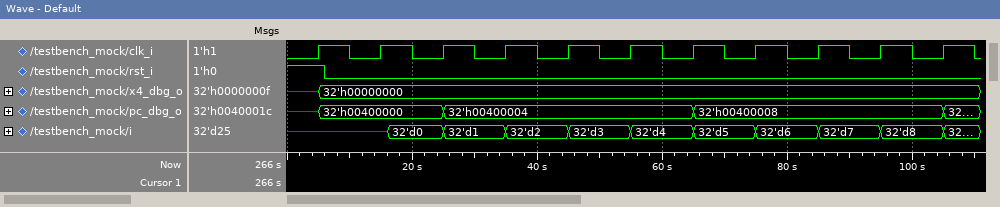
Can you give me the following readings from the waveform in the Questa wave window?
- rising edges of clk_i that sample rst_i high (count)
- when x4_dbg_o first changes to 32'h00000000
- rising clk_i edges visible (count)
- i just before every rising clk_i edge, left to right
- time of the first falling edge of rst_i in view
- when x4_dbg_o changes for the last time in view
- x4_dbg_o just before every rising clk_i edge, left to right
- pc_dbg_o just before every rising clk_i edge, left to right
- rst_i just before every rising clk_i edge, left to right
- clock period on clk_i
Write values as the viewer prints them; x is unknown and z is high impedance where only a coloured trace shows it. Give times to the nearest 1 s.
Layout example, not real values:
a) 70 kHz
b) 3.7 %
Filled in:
a) 1
b) 5 s
c) 11
d) x, x, 32'd0, 32'd1, 32'd2, 32'd3, 32'd4, 32'd5, 32'd6, 32'd7, 32'd8
e) 6 s
f) 5 s
g) x, 32'h00000000, 32'h00000000, 32'h00000000, 32'h00000000, 32'h00000000, 32'h00000000, 32'h00000000, 32'h00000000, 32'h00000000, 32'h00000000
h) x, 32'h00400000, 32'h00400000, 32'h00400004, 32'h00400004, 32'h00400004, 32'h00400004, 32'h00400008, 32'h00400008, 32'h00400008, 32'h00400008
i) 1 0 0 0 0 0 0 0 0 0 0
j) 10 s
